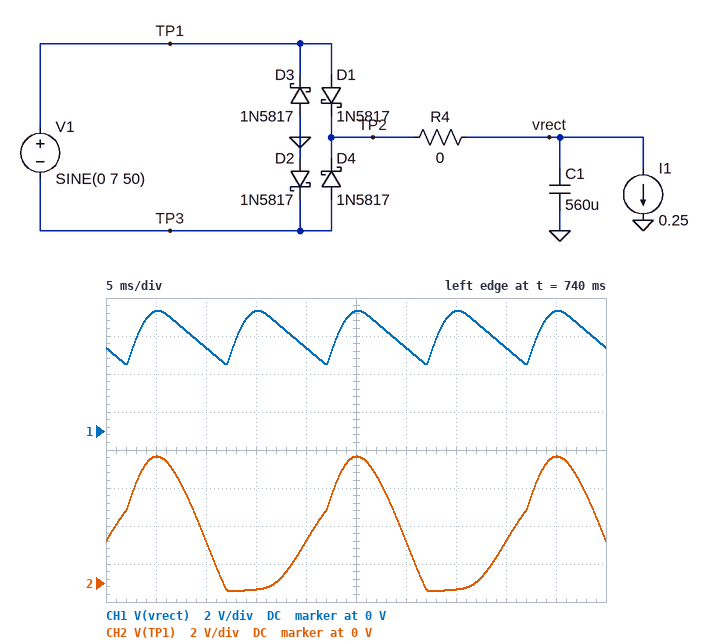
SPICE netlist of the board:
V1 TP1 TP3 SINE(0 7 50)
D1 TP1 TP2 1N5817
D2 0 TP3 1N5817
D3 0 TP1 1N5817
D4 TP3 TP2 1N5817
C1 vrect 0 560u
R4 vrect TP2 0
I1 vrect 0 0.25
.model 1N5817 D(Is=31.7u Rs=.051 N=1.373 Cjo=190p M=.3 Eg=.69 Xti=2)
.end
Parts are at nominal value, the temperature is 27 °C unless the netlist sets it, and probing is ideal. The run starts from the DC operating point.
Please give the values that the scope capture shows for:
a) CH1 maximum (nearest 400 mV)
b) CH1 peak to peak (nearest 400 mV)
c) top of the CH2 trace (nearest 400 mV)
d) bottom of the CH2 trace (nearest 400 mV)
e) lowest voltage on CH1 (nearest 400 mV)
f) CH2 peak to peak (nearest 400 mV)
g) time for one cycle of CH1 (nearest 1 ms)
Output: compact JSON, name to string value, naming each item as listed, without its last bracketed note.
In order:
{"CH1 maximum": "6.4 V", "CH1 peak to peak": "2.8 V", "top of the CH2 trace": "6.8 V", "bottom of the CH2 trace": "-400 mV", "lowest voltage on CH1": "3.6 V", "CH2 peak to peak": "7.2 V", "time for one cycle of CH1": "10 ms"}
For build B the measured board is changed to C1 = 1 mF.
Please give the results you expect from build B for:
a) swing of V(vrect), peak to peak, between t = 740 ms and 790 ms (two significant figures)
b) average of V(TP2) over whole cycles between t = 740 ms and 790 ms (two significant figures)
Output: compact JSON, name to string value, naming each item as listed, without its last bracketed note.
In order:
{"swing of V(vrect), peak to peak, between t = 740 ms and 790 ms": "1.8 V", "average of V(TP2) over whole cycles between t = 740 ms and 790 ms": "5.5 V"}
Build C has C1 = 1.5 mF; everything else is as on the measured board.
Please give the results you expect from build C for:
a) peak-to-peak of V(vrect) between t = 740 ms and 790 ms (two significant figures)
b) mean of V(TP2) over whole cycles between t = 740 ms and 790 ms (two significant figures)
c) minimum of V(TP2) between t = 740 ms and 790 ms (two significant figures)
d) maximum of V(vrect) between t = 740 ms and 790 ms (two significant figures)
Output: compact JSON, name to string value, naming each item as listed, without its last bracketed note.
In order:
{"peak-to-peak of V(vrect) between t = 740 ms and 790 ms": "1.2 V", "mean of V(TP2) over whole cycles between t = 740 ms and 790 ms": "5.7 V", "minimum of V(TP2) between t = 740 ms and 790 ms": "5.1 V", "maximum of V(vrect) between t = 740 ms and 790 ms": "6.3 V"}
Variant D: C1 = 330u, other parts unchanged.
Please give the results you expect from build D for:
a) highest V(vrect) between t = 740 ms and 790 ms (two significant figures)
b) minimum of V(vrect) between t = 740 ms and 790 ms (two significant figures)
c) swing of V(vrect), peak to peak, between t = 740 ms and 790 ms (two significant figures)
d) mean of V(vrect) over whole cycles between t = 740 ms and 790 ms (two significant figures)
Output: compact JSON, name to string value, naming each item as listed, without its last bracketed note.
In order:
{"highest V(vrect) between t = 740 ms and 790 ms": "6.3 V", "minimum of V(vrect) between t = 740 ms and 790 ms": "2.2 V", "swing of V(vrect), peak to peak, between t = 740 ms and 790 ms": "4.2 V", "mean of V(vrect) over whole cycles between t = 740 ms and 790 ms": "4.6 V"}
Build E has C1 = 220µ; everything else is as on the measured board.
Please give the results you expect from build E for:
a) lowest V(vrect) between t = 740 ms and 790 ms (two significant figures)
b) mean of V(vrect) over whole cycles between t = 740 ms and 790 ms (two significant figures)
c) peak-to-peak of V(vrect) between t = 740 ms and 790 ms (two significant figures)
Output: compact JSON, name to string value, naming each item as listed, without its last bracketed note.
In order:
{"lowest V(vrect) between t = 740 ms and 790 ms": "1.0 V", "mean of V(vrect) over whole cycles between t = 740 ms and 790 ms": "4.2 V", "peak-to-peak of V(vrect) between t = 740 ms and 790 ms": "5.3 V"}
